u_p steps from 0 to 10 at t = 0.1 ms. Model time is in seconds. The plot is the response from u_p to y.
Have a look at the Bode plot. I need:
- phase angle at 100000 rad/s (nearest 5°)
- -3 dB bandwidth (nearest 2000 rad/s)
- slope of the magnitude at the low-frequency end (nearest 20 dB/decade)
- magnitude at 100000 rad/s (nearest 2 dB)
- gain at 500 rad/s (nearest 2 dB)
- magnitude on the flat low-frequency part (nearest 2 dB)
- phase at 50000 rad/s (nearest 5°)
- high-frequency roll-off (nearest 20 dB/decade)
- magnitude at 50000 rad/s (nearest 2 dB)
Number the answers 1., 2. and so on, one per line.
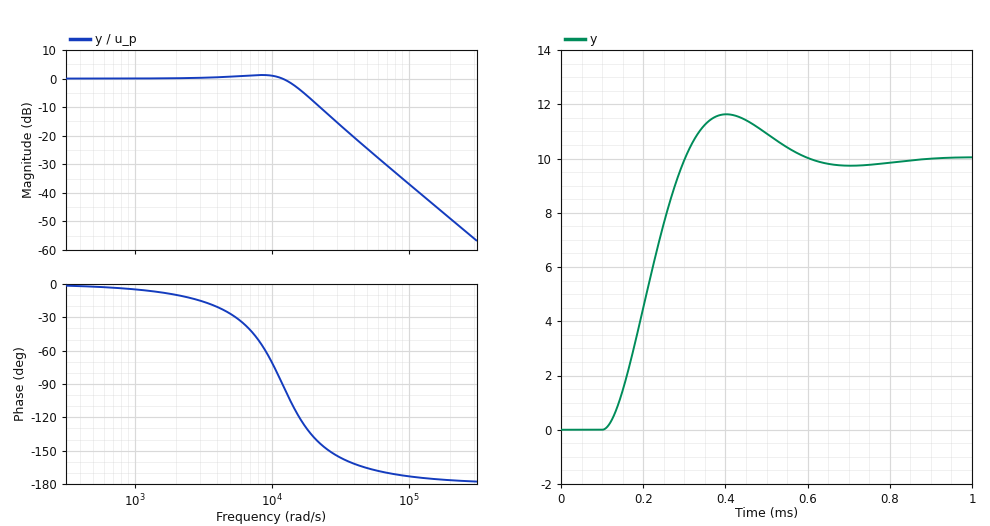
1. -175°
2. 16000 rad/s
3. 0 dB/decade
4. -36 dB
5. 0 dB
6. 0 dB
7. -165°
8. -40 dB/decade
9. -24 dB
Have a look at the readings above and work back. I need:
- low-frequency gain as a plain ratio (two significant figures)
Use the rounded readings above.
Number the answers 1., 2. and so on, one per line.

1. 1.0
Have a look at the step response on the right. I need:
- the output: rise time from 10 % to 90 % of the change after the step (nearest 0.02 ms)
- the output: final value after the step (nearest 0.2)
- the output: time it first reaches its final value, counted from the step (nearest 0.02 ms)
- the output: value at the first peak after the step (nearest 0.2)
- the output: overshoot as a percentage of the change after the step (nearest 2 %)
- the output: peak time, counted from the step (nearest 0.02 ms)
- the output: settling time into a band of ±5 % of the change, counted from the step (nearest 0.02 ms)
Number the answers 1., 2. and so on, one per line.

1. 0.14 ms
2. 10.0
3. 0.20 ms
4. 11.6
5. 16 %
6. 0.30 ms
7. 0.44 ms
